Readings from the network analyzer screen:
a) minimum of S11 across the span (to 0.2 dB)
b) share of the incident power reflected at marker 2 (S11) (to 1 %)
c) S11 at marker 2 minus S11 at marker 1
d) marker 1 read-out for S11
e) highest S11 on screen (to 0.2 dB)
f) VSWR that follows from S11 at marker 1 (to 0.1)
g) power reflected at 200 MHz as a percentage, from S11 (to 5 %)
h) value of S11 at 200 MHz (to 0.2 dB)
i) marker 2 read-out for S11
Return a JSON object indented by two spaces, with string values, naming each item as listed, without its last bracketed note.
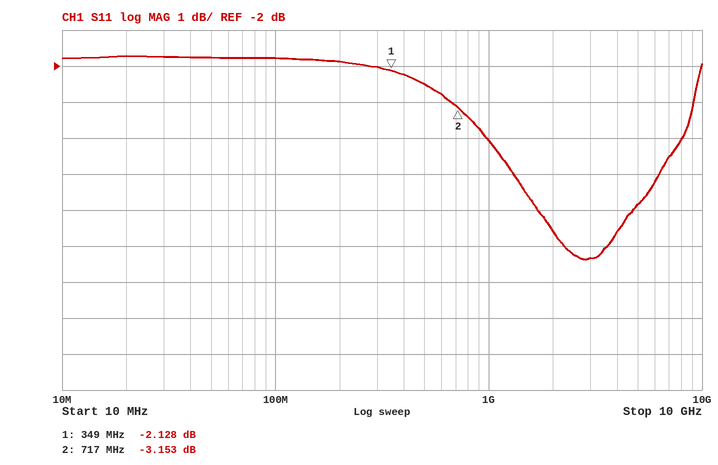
{
  "minimum of S11 across the span": "-7.4 dB",
  "share of the incident power reflected at marker 2 (S11)": "48 %",
  "S11 at marker 2 minus S11 at marker 1": "-1.025 dB",
  "marker 1 read-out for S11": "-2.128 dB",
  "highest S11 on screen": "-1.8 dB",
  "VSWR that follows from S11 at marker 1": "8.2",
  "power reflected at 200 MHz as a percentage, from S11": "65 %",
  "value of S11 at 200 MHz": "-1.8 dB",
  "marker 2 read-out for S11": "-3.153 dB"
}
